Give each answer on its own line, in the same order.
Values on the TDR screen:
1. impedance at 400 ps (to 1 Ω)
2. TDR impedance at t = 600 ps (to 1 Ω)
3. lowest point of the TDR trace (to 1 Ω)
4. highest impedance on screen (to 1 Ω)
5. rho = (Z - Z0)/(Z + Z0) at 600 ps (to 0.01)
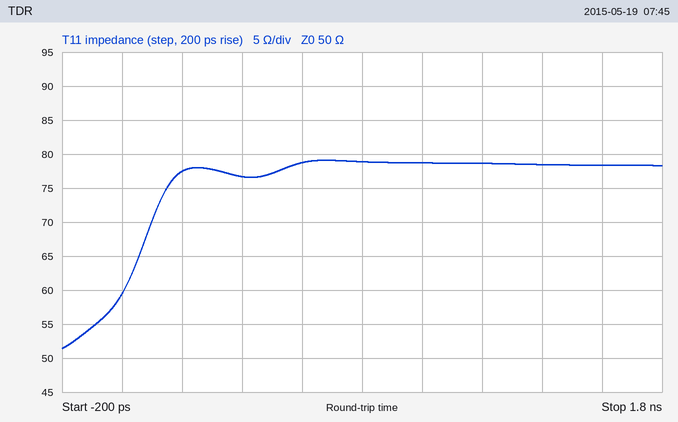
77 Ω
79 Ω
51 Ω
79 Ω
+0.22
